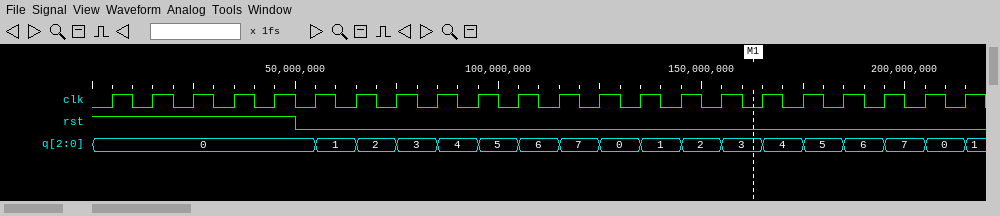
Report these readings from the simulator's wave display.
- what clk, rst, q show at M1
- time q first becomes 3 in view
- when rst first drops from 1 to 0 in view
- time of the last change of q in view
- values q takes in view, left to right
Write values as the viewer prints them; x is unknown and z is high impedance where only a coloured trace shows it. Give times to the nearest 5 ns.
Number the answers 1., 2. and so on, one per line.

1. clk=0, rst=0, q=3
2. 75 ns
3. 50 ns
4. 215 ns
5. 0, 1, 2, 3, 4, 5, 6, 7, 0, 1, 2, 3, 4, 5, 6, 7, 0, 1
